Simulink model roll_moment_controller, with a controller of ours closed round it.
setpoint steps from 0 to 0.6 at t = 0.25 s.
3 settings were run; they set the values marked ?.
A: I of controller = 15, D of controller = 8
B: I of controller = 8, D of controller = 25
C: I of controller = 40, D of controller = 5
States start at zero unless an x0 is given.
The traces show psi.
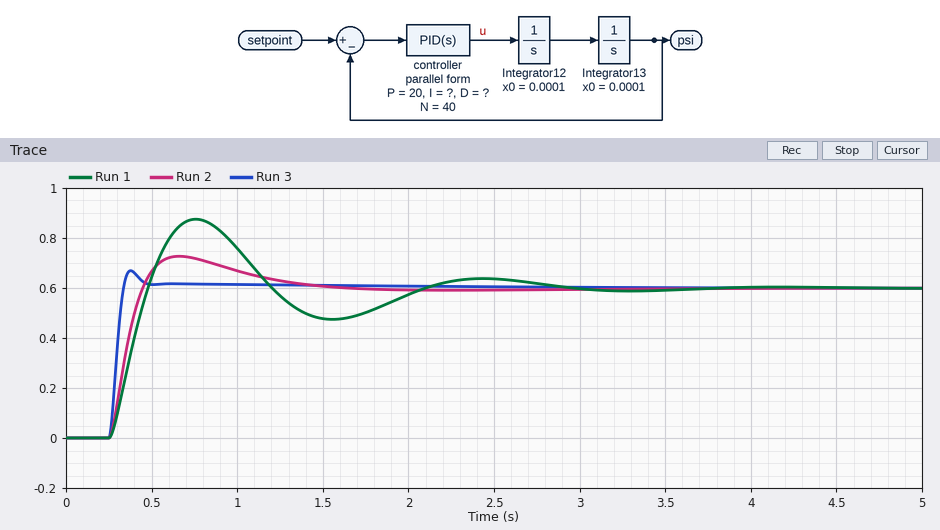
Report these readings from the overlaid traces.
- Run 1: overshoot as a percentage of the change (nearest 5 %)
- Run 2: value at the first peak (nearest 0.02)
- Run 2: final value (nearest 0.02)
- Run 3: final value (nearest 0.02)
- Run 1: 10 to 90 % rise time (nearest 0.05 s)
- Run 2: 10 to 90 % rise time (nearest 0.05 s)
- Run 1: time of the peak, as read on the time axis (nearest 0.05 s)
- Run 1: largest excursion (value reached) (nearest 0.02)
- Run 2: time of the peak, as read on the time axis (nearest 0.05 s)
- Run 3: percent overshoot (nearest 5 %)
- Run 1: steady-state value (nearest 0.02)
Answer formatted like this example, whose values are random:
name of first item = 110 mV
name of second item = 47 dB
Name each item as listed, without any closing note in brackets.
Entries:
Run 1: overshoot as a percentage of the change = 45 %
Run 2: value at the first peak = 0.72
Run 2: final value = 0.60
Run 3: final value = 0.60
Run 1: 10 to 90 % rise time = 0.15 s
Run 2: 10 to 90 % rise time = 0.15 s
Run 1: time of the peak, as read on the time axis = 0.75 s
Run 1: largest excursion (value reached) = 0.88
Run 2: time of the peak, as read on the time axis = 0.65 s
Run 3: percent overshoot = 10 %
Run 1: steady-state value = 0.60
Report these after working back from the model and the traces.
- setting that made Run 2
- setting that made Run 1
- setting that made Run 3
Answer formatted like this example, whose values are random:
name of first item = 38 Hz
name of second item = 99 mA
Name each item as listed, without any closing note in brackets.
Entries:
setting that made Run 2 = A
setting that made Run 1 = C
setting that made Run 3 = B
